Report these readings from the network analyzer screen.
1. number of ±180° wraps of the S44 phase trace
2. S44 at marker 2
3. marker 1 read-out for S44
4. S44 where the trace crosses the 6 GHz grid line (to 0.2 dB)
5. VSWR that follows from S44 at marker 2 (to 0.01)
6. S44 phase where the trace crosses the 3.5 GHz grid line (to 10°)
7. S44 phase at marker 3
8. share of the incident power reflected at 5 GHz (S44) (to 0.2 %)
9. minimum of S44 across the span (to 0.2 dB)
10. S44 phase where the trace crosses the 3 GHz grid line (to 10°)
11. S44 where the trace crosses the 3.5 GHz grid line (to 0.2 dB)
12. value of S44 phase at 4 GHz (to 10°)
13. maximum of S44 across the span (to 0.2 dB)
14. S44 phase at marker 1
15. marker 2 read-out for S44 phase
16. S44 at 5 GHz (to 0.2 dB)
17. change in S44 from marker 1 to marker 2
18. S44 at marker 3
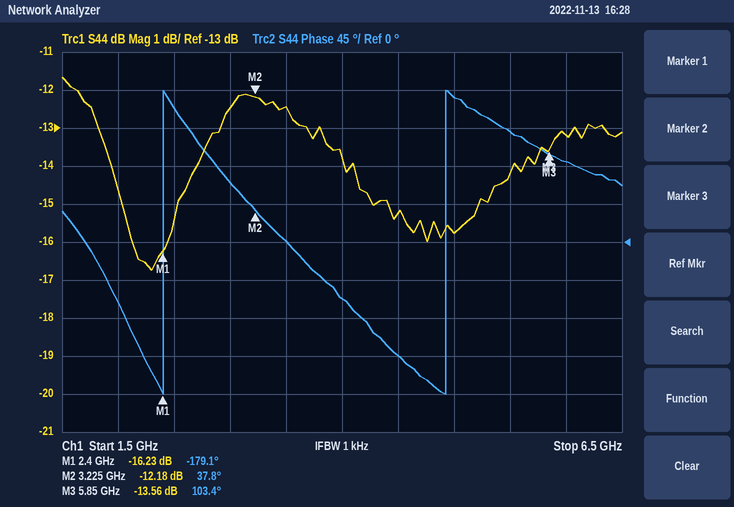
2
-12.18 dB
-16.23 dB
-13.2 dB
1.65
0°
103.4°
2.6 %
-16.8 dB
70°
-12.4 dB
-70°
-11.6 dB
-179.1°
37.8°
-15.8 dB
4.05 dB
-13.56 dB
